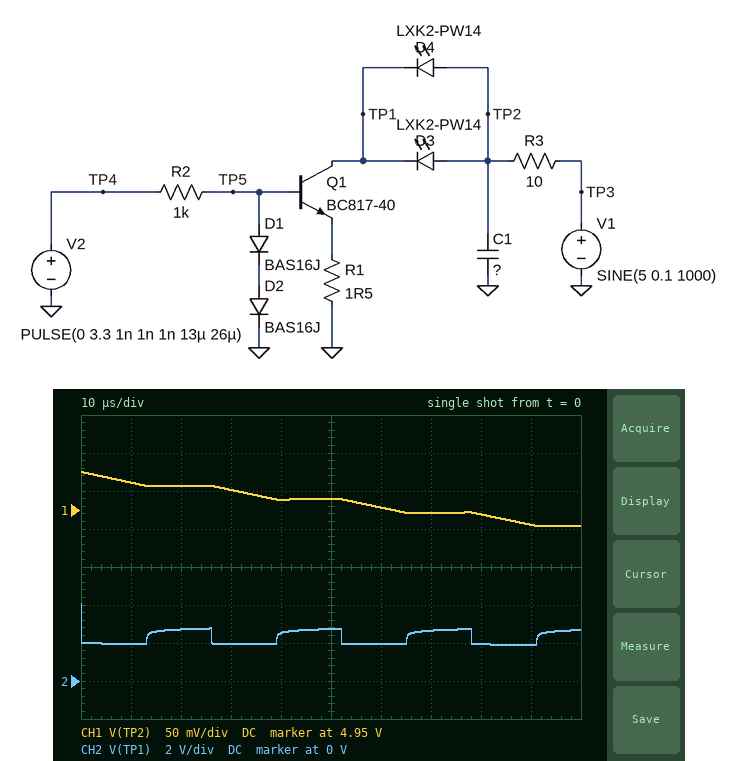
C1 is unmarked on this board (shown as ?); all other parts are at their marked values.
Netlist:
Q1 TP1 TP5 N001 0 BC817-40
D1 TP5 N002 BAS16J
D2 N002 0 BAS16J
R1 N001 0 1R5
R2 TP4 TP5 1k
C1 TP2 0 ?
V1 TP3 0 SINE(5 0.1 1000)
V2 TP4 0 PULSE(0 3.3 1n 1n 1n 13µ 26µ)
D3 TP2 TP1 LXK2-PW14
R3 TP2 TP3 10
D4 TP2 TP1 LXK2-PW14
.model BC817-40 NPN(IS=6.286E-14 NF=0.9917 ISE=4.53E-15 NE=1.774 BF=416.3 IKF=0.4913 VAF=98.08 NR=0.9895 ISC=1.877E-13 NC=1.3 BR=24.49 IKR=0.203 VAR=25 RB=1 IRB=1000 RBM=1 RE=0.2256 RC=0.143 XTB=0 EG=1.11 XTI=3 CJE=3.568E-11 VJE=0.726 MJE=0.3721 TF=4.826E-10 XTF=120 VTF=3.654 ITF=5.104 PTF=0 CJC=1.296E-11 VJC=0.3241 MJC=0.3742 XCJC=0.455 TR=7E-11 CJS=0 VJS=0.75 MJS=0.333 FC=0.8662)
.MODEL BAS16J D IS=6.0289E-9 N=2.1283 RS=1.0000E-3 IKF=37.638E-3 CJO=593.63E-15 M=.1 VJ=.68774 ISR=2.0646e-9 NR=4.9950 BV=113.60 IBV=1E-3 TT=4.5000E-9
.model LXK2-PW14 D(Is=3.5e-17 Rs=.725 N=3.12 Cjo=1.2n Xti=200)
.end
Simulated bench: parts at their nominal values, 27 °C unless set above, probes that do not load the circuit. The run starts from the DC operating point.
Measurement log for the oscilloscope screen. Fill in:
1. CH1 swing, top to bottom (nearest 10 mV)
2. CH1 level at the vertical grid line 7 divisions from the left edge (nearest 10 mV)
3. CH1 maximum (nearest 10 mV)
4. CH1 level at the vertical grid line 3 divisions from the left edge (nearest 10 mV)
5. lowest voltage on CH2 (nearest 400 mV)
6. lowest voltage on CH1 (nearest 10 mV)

70 mV
4.95 V
5.00 V
4.98 V
2.0 V
4.93 V
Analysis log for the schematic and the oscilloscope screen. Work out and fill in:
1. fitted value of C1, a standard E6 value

220 µF
